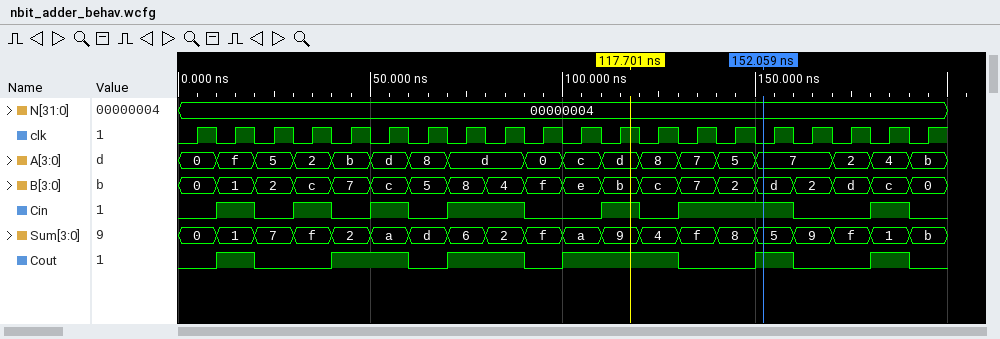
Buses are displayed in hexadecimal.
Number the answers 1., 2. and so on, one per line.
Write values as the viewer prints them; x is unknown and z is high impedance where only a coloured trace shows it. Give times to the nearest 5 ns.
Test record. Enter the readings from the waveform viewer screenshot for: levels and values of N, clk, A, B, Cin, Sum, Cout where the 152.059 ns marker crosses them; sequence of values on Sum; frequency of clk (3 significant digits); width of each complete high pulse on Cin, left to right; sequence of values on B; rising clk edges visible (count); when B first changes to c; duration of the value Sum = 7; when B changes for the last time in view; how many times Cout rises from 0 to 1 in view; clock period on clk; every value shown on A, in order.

1. N=00000004, clk=0, A=7, B=d, Cin=1, Sum=5, Cout=1
2. 0, 1, 7, f, 2, a, d, 6, 2, f, a, 9, 4, f, 8, 5, 9, f, 1, b
3. 100 MHz
4. 10 ns, 10 ns, 10 ns, 20 ns, 10 ns, 30 ns, 10 ns
5. 0, 1, 2, c, 7, c, 5, 8, 4, f, e, b, c, 7, 2, d, 2, d, c, 0
6. 20
7. 30 ns
8. 10 ns
9. 190 ns
10. 6
11. 10 ns
12. 0, f, 5, 2, b, d, 8, d, 0, c, d, 8, 7, 5, 7, 2, 4, b
